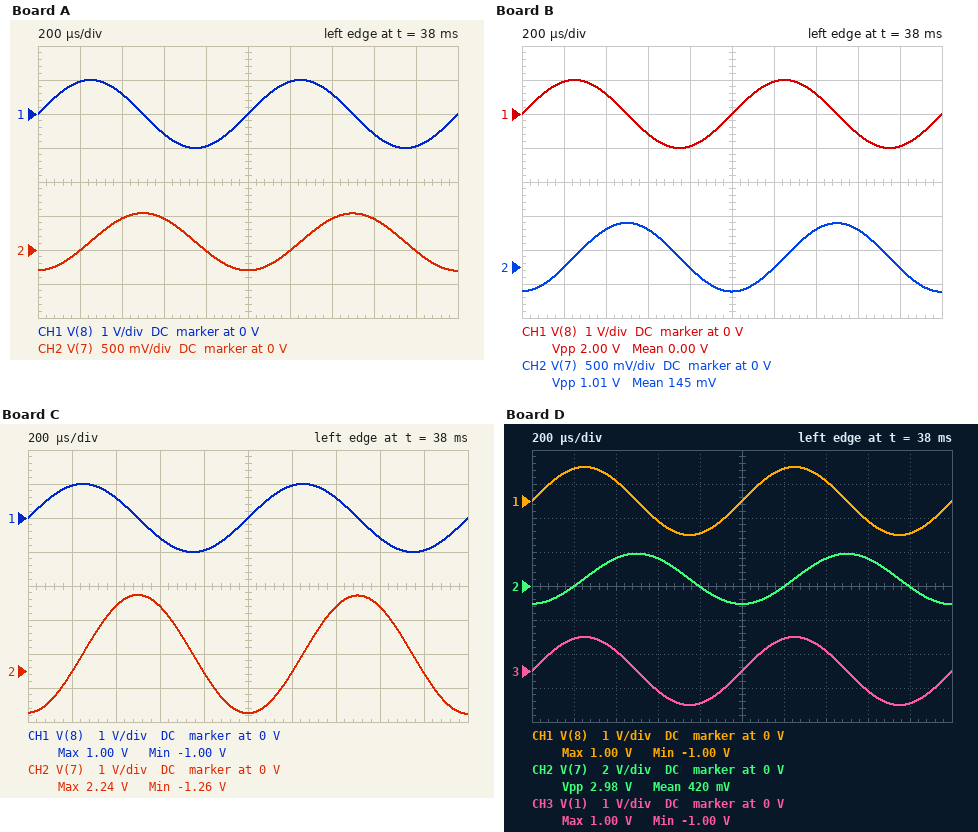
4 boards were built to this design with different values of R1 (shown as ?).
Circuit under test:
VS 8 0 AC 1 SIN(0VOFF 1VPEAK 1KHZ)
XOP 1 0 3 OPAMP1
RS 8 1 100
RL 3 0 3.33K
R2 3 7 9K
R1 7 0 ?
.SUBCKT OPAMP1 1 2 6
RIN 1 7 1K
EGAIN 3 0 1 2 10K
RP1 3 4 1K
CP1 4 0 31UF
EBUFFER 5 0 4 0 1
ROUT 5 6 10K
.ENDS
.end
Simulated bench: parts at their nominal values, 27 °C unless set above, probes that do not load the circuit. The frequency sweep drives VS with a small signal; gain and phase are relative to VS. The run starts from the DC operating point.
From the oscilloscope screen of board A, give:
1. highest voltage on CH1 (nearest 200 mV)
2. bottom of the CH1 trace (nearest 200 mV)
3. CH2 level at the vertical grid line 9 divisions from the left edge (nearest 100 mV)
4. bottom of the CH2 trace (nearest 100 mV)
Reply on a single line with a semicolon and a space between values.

1.0 V; -1.0 V; 0 V; -300 mV
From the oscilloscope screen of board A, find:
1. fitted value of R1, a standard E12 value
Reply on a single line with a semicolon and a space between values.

390 Ω
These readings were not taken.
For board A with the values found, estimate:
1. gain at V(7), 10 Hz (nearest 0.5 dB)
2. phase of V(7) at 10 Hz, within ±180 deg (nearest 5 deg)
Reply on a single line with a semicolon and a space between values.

31.5 dB; -65 deg
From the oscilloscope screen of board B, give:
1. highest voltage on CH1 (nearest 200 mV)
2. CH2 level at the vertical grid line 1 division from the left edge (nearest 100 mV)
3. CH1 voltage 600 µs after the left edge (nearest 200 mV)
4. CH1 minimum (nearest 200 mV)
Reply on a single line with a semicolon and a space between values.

1.0 V; 0 V; -600 mV; -1.0 V
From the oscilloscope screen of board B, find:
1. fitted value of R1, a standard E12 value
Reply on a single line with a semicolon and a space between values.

470 Ω
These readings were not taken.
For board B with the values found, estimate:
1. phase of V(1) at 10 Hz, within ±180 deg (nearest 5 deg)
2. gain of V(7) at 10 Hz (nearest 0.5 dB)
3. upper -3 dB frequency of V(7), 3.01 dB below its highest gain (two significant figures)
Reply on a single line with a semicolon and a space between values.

0 deg; 33.0 dB; 5.1 Hz
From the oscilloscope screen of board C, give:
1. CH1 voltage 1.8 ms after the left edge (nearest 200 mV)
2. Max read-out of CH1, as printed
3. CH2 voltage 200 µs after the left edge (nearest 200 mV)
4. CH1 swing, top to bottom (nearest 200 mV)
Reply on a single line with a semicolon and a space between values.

-1.0 V; 1.00 V; 0 V; 2.0 V
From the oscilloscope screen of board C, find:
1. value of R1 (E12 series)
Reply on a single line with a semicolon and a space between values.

1.8 kΩ
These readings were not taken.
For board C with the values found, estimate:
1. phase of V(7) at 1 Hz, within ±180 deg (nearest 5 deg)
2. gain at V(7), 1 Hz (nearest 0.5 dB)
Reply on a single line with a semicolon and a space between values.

-10 deg; 50.5 dB
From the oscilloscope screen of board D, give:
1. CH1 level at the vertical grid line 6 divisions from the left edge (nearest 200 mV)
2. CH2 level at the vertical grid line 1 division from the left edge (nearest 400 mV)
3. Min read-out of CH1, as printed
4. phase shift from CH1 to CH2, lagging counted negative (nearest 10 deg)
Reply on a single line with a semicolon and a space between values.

1.0 V; 0 V; -1.00 V; -90 deg
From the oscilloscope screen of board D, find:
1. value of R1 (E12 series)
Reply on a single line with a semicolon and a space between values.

1.5 kΩ
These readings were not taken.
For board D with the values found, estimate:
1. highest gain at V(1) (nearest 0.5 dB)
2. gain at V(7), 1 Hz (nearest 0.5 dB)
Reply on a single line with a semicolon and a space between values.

0 dB; 49.0 dB
